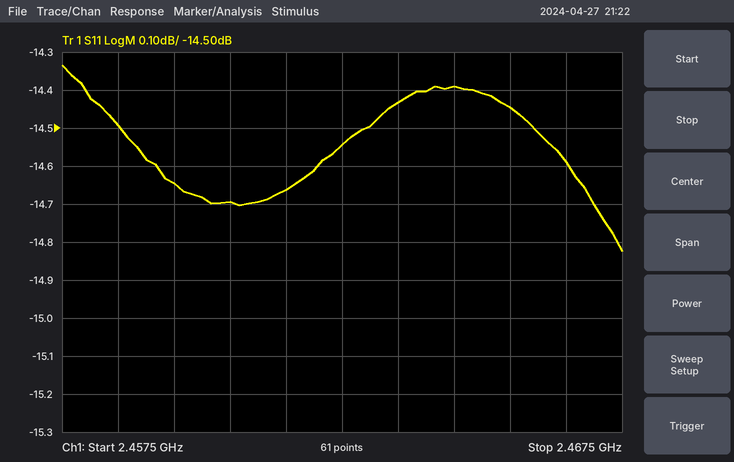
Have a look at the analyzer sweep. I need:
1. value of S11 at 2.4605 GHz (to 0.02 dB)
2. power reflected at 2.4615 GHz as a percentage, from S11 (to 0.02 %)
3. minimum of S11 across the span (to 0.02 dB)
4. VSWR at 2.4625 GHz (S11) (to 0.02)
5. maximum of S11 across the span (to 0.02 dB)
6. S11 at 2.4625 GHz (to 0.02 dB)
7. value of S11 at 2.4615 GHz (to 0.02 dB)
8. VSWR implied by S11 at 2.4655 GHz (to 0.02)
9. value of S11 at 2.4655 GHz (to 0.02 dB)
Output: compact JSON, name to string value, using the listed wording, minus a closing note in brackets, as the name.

{"value of S11 at 2.4605 GHz": "-14.70 dB", "power reflected at 2.4615 GHz as a percentage, from S11": "3.42 %", "minimum of S11 across the span": "-14.82 dB", "VSWR at 2.4625 GHz (S11)": "1.46", "maximum of S11 across the span": "-14.34 dB", "S11 at 2.4625 GHz": "-14.54 dB", "value of S11 at 2.4615 GHz": "-14.66 dB", "VSWR implied by S11 at 2.4655 GHz": "1.46", "value of S11 at 2.4655 GHz": "-14.44 dB"}
